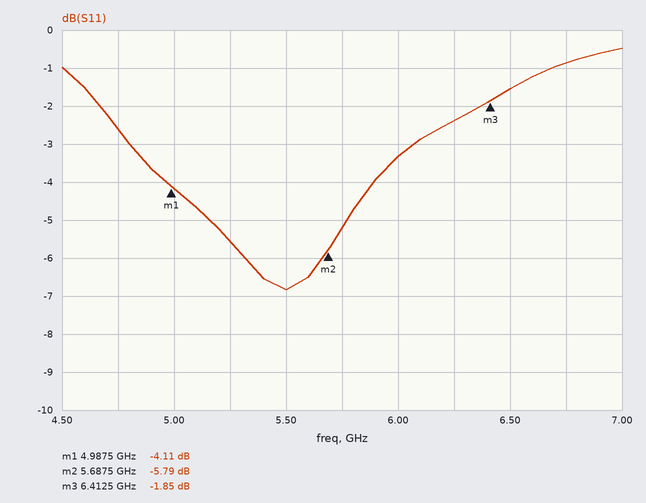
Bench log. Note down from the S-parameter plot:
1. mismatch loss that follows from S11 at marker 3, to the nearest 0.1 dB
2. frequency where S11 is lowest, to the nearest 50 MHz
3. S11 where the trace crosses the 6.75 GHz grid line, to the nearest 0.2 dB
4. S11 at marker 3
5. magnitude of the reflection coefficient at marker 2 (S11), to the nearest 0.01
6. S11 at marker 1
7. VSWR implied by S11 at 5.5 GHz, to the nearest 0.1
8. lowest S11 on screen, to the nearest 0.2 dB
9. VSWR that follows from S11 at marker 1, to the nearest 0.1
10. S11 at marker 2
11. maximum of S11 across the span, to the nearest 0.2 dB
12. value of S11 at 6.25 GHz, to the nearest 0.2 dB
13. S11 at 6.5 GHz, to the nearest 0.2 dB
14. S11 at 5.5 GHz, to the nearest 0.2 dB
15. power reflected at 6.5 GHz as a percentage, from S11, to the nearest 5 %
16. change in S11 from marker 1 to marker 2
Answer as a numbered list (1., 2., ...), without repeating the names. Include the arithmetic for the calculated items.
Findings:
1. −10 log10(1 − 10^(-1.85/10)) ≈ 4.6 dB
2. 5.50 GHz
3. -0.8 dB
4. -1.85 dB
5. 10^(-5.79/20) ≈ 0.51
6. -4.11 dB
7. |Γ| = 10^(-6.8/20) = 0.4571; VSWR = (1 + 0.4571)/(1 − 0.4571) ≈ 2.7
8. -6.8 dB
9. (1 + 0.6230)/(1 − 0.6230) ≈ 4.3
10. -5.79 dB
11. -0.4 dB
12. -2.4 dB
13. -1.6 dB
14. -6.8 dB
15. 10^(-1.6/10) ≈ 69.2 %, so 70 % to the nearest 5 %
16. -5.79 − (-4.11) = -1.68 dB
